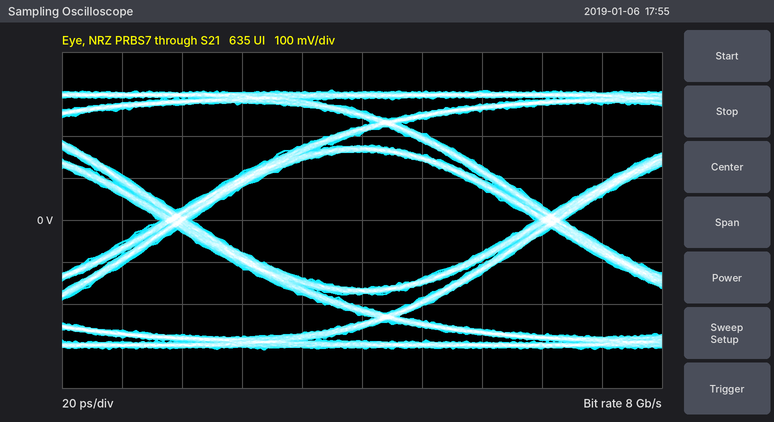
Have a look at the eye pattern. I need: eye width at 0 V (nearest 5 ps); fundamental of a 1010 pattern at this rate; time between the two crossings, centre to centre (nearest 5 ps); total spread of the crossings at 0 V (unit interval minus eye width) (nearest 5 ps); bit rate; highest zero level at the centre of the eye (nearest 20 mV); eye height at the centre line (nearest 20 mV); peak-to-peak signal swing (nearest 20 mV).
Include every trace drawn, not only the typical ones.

115 ps
4 GHz
125 ps
10 ps
8 Gb/s
-160 mV
320 mV
620 mV
